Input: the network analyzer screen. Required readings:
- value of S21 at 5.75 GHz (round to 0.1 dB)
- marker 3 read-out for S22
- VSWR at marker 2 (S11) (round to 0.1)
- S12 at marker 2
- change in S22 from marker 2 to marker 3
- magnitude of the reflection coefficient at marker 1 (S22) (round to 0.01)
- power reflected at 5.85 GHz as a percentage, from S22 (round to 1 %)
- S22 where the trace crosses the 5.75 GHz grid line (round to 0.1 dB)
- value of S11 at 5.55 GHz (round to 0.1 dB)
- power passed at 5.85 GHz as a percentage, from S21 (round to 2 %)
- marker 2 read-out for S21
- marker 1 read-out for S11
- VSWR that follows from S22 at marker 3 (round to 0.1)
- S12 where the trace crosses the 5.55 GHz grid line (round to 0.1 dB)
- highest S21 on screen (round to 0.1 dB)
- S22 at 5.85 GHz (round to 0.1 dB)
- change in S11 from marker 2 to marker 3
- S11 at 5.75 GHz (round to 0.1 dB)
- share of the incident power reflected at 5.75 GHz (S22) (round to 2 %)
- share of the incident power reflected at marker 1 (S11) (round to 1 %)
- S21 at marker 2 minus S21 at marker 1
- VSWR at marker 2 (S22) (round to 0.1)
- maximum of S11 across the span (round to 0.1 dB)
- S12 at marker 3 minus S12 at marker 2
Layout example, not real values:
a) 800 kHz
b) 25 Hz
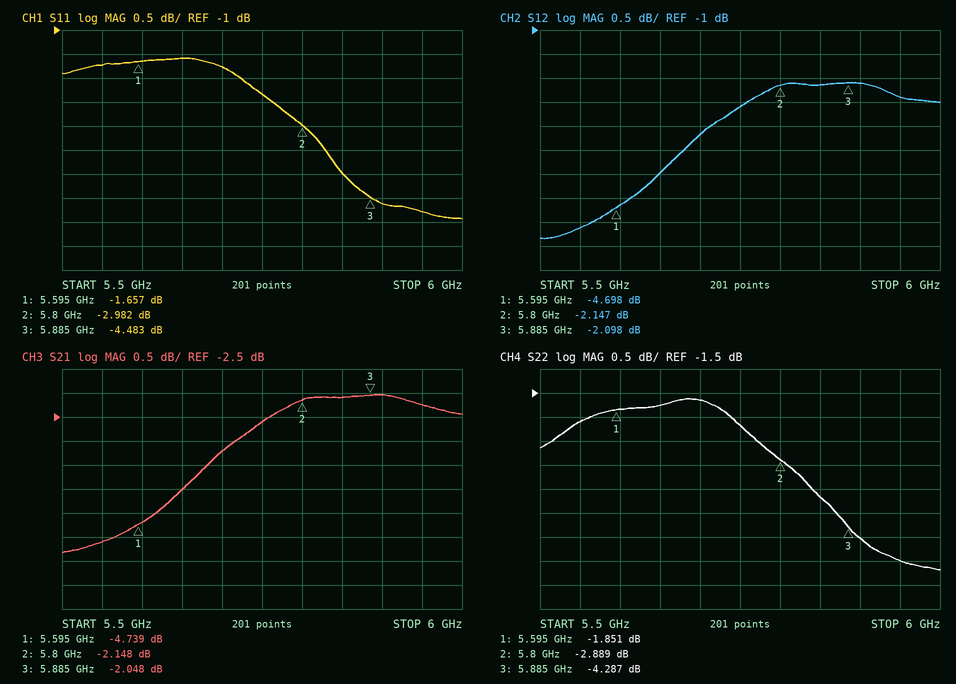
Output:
a) -2.6 dB
b) -4.287 dB
c) 5.9
d) -2.147 dB
e) -1.398 dB
f) 0.81
g) 43 %
h) -2.2 dB
i) -1.7 dB
j) 62 %
k) -2.148 dB
l) -1.657 dB
m) 4.1
n) -5.1 dB
o) -2.0 dB
p) -3.7 dB
q) -1.501 dB
r) -2.3 dB
s) 60 %
t) 68 %
u) 2.591 dB
v) 6.1
w) -1.6 dB
x) 0.049 dB
